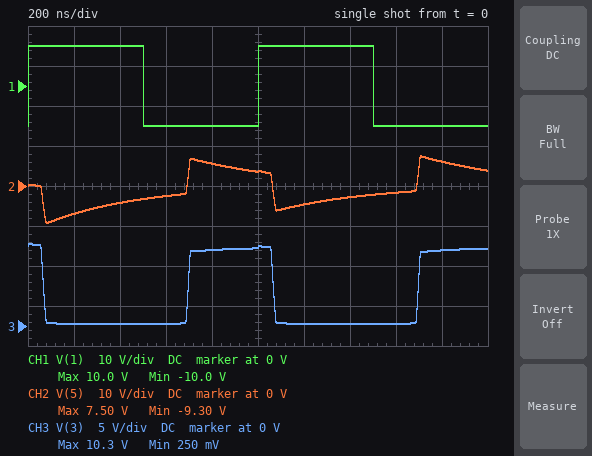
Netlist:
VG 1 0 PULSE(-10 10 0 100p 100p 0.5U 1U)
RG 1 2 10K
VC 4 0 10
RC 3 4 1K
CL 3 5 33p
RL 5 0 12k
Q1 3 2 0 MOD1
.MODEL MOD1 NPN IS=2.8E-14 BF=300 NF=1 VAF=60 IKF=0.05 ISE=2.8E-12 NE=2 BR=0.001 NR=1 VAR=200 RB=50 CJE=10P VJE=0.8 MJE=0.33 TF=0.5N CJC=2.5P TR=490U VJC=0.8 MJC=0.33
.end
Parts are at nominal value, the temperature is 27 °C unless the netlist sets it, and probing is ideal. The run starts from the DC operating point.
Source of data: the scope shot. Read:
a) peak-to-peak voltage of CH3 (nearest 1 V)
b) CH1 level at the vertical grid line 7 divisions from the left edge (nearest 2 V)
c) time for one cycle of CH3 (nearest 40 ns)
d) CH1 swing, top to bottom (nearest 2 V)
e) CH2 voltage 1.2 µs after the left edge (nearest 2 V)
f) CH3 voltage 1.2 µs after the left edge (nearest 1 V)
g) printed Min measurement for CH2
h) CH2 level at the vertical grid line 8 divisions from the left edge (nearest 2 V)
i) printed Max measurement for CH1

10 V
10 V
1.00 µs
20 V
-4 V
0 V
-9.30 V
-2 V
10.0 V
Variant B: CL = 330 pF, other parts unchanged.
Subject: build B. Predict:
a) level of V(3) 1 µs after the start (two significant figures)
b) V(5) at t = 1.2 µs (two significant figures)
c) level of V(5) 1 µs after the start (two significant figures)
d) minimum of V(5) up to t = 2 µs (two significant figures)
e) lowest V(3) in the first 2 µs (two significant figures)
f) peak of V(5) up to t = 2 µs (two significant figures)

9.9 V
-8.1 V
1.2 V
-9.6 V
260 mV
2.3 V
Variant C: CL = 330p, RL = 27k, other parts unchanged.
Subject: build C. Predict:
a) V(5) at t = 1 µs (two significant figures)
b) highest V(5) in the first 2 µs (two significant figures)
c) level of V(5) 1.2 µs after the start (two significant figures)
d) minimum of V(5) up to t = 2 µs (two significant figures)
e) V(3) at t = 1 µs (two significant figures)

620 mV
1.2 V
-8.9 V
-9.6 V
10 V
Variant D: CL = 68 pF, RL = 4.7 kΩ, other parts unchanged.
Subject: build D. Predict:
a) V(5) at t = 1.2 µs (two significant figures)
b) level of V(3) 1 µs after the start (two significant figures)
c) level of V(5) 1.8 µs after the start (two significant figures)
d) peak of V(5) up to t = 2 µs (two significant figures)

-4.3 V
9.3 V
5.5 V
7.0 V
